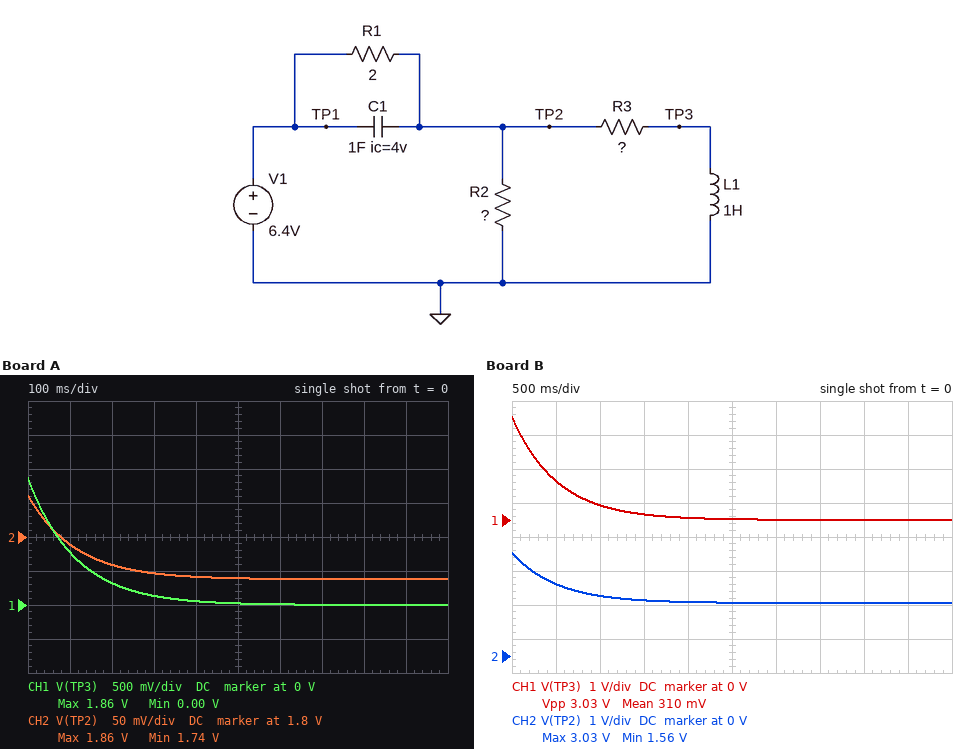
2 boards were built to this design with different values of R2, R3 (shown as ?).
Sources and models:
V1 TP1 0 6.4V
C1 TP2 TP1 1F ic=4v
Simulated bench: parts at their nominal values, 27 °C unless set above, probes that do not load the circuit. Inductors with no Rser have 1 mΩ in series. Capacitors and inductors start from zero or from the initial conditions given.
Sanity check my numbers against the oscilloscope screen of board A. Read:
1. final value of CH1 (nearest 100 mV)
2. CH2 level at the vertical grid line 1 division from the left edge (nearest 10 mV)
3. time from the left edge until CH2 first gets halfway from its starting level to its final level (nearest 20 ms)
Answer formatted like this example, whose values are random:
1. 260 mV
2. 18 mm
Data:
1. 0 V
2. 1.79 V
3. 80 ms
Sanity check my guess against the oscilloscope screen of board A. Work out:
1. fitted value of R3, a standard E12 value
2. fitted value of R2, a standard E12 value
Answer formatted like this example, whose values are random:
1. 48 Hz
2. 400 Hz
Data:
1. 8.2 Ω
2. 0.82 Ω
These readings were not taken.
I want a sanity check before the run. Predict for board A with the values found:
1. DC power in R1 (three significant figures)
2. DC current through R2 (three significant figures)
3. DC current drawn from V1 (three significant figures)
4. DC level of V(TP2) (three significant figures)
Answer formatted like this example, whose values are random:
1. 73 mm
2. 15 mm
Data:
1. 10.9 W
2. 2.12 A
3. 2.33 A
4. 1.74 V
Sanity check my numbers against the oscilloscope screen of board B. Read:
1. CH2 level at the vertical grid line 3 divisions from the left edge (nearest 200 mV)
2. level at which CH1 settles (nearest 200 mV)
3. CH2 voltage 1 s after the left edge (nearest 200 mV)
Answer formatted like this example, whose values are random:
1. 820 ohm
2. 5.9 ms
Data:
1. 1.6 V
2. 0 V
3. 1.8 V
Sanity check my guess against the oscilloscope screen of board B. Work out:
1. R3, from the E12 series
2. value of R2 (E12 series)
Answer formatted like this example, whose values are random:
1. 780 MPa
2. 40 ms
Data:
1. 1 Ω
2. 1.8 Ω
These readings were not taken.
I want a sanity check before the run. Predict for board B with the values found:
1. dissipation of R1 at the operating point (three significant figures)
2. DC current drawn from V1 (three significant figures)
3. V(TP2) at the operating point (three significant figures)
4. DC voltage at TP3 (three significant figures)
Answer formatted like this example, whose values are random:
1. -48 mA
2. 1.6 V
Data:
1. 11.7 W
2. 2.42 A
3. 1.56 V
4. 1.56 mV
